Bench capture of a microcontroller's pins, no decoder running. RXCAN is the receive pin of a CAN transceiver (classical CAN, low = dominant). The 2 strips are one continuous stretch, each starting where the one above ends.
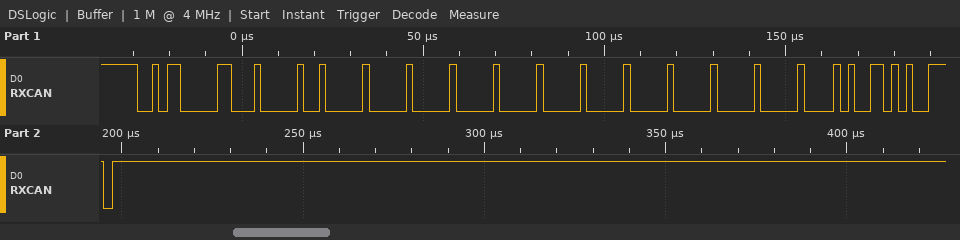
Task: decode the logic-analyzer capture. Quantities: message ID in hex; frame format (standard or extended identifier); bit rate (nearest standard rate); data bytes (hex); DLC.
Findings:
0x2C1
standard
500 kbit/s
08 00 00 00 00 00 00 00
8
